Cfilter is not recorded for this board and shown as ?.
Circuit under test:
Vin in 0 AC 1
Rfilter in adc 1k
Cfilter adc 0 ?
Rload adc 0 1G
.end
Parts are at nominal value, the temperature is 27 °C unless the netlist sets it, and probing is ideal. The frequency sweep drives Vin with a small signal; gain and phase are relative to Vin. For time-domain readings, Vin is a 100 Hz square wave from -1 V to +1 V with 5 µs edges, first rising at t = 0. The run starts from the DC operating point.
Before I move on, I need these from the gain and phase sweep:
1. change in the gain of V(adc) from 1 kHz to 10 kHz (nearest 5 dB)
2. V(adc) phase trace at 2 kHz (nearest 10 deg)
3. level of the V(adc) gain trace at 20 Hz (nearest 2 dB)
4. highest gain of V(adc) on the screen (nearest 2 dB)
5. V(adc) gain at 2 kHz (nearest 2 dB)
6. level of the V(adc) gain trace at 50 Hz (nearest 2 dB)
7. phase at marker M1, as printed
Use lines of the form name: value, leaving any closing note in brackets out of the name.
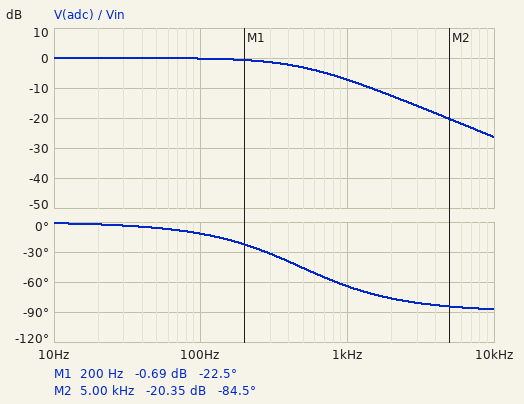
change in the gain of V(adc) from 1 kHz to 10 kHz: -20 dB
V(adc) phase trace at 2 kHz: -80 deg
level of the V(adc) gain trace at 20 Hz: 0 dB
highest gain of V(adc) on the screen: 0 dB
V(adc) gain at 2 kHz: -12 dB
level of the V(adc) gain trace at 50 Hz: 0 dB
phase at marker M1, as printed: -22.5 deg
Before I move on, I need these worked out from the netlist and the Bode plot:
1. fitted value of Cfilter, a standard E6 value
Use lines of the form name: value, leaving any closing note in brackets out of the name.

fitted value of Cfilter, a standard E6 value: 330 nF
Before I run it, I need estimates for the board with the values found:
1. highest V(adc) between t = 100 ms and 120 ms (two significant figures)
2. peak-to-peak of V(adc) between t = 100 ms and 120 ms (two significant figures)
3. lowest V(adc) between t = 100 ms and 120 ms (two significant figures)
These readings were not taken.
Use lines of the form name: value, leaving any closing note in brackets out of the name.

highest V(adc) between t = 100 ms and 120 ms: 1.0 V
peak-to-peak of V(adc) between t = 100 ms and 120 ms: 2.0 V
lowest V(adc) between t = 100 ms and 120 ms: -1.0 V
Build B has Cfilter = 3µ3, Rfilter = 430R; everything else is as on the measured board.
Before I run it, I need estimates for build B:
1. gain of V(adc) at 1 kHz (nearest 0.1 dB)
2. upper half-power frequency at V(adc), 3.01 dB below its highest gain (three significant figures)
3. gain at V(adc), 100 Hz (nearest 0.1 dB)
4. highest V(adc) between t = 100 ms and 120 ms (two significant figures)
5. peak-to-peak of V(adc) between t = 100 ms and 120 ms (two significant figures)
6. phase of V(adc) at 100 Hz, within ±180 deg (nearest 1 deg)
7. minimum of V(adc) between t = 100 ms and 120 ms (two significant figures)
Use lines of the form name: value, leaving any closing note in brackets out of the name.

gain of V(adc) at 1 kHz: -19.1 dB
upper half-power frequency at V(adc), 3.01 dB below its highest gain: 112 Hz
gain at V(adc), 100 Hz: -2.5 dB
highest V(adc) between t = 100 ms and 120 ms: 940 mV
peak-to-peak of V(adc) between t = 100 ms and 120 ms: 1.9 V
phase of V(adc) at 100 Hz, within ±180 deg: -42 deg
minimum of V(adc) between t = 100 ms and 120 ms: -940 mV
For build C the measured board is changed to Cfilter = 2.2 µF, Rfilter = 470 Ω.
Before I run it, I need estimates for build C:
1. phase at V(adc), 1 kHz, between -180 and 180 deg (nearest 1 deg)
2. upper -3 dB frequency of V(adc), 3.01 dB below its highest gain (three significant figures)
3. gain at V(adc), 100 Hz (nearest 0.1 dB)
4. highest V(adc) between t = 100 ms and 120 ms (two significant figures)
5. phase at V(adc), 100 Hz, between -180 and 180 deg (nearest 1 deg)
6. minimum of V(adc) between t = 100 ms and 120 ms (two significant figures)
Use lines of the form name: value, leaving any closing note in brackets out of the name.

phase at V(adc), 1 kHz, between -180 and 180 deg: -81 deg
upper -3 dB frequency of V(adc), 3.01 dB below its highest gain: 154 Hz
gain at V(adc), 100 Hz: -1.5 dB
highest V(adc) between t = 100 ms and 120 ms: 980 mV
phase at V(adc), 100 Hz, between -180 and 180 deg: -33 deg
minimum of V(adc) between t = 100 ms and 120 ms: -980 mV
